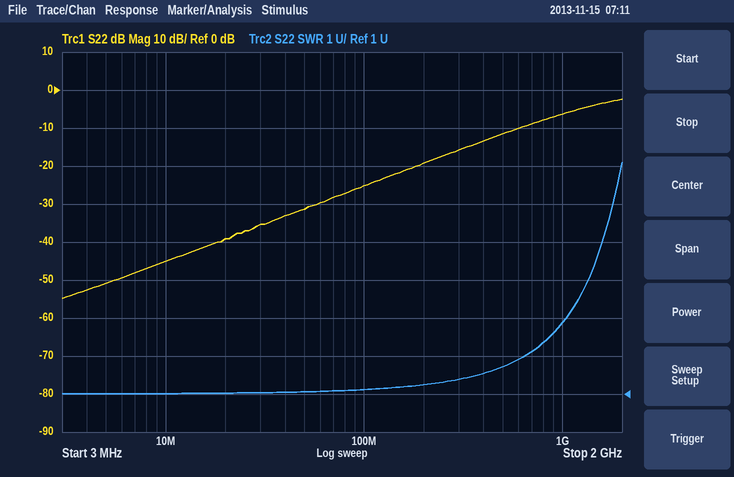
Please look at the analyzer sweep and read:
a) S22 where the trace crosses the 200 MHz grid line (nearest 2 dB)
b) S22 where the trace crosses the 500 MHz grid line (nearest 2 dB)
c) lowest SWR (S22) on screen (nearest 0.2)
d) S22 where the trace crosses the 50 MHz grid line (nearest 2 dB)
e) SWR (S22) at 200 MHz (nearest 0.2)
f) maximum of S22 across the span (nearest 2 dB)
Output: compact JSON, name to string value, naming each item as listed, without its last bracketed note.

{"S22 where the trace crosses the 200 MHz grid line": "-20 dB", "S22 where the trace crosses the 500 MHz grid line": "-12 dB", "lowest SWR (S22) on screen": "1.0", "S22 where the trace crosses the 50 MHz grid line": "-32 dB", "SWR (S22) at 200 MHz": "1.2", "maximum of S22 across the span": "-2 dB"}
